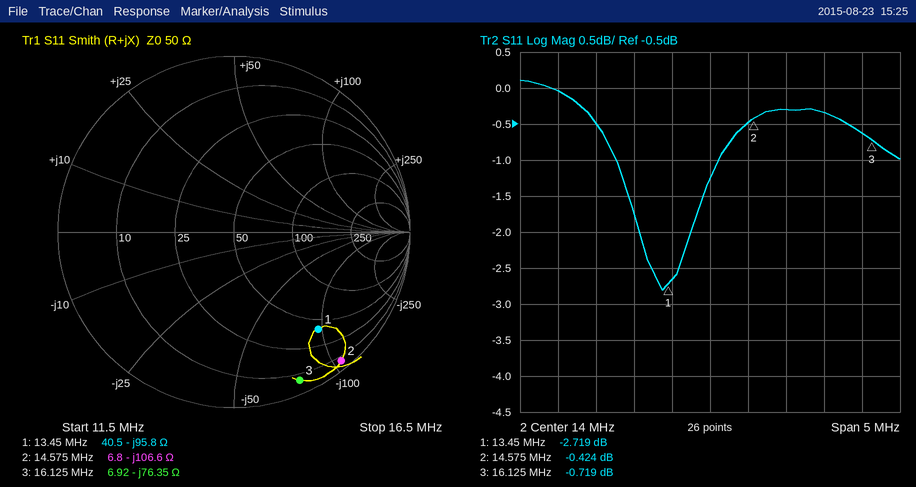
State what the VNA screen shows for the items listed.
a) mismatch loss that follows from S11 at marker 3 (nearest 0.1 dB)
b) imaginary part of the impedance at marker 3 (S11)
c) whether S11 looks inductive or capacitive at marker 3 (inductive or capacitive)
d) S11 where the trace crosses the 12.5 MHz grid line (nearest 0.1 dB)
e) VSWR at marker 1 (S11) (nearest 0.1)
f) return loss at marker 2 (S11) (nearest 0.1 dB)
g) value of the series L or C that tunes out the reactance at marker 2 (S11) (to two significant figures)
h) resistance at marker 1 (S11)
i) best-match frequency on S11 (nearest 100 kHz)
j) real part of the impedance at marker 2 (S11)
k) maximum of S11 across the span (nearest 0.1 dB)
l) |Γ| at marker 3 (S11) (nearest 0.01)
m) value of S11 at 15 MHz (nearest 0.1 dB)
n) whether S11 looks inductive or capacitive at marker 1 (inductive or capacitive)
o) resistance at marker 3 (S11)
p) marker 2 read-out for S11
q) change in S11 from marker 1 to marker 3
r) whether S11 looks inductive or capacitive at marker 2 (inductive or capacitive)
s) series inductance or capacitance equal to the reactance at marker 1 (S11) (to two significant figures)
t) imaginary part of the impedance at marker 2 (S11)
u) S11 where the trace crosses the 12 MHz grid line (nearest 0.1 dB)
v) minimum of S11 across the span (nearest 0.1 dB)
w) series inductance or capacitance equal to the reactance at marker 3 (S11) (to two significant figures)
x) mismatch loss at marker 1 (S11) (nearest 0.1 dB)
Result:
8.2 dB
-76.35 Ω
capacitive
-0.5 dB
6.4
0.4 dB
1.2 µH
40.5 Ω
13.4 MHz
6.8 Ω
0.1 dB
0.92
-0.3 dB
capacitive
6.92 Ω
-0.424 dB
2.000 dB
capacitive
120 pF
-106.6 Ω
0.0 dB
-2.8 dB
130 pF
3.3 dB
